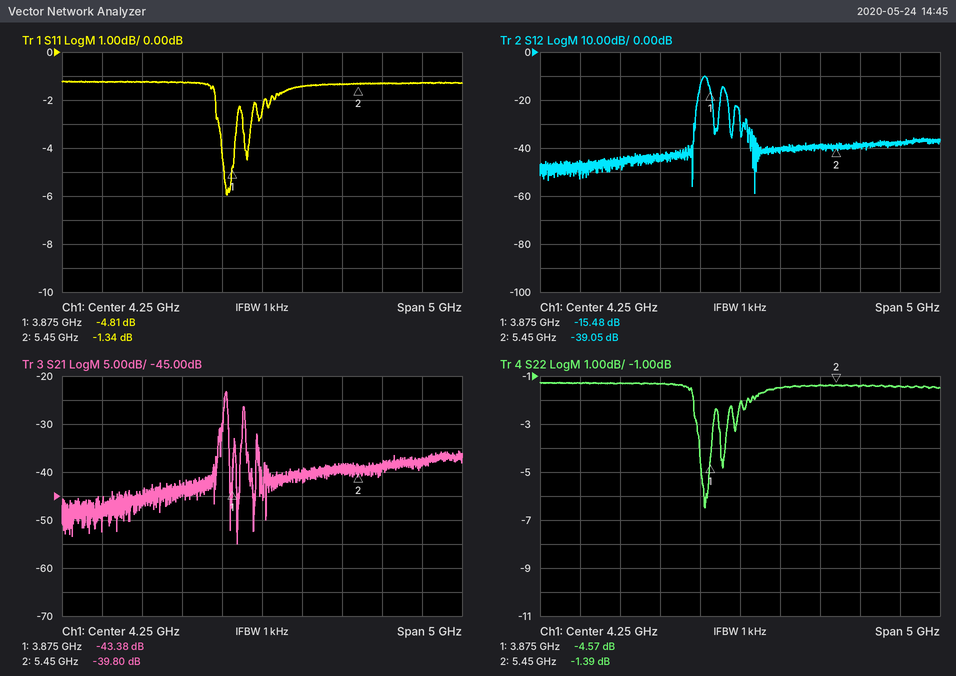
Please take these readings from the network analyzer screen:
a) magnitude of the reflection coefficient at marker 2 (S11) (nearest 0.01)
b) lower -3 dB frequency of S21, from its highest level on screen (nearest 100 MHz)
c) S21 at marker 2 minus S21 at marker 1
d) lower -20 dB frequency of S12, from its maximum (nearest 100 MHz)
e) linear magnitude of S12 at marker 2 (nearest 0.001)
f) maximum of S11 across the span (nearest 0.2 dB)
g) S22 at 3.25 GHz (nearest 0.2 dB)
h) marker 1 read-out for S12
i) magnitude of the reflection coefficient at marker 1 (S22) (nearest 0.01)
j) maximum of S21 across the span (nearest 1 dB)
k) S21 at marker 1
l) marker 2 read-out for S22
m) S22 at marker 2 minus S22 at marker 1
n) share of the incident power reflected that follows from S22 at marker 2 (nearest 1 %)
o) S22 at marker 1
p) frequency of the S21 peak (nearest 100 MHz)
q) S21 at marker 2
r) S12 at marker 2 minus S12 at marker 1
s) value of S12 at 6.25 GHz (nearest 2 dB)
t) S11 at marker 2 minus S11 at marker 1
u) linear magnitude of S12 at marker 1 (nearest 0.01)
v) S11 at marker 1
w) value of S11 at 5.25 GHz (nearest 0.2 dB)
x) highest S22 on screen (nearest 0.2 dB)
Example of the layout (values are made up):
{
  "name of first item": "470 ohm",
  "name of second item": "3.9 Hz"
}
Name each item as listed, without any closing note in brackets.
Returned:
{
  "magnitude of the reflection coefficient at marker 2 (S11)": "0.86",
  "lower -3 dB frequency of S21, from its highest level on screen": "3.8 GHz",
  "S21 at marker 2 minus S21 at marker 1": "3.58 dB",
  "lower -20 dB frequency of S12, from its maximum": "3.7 GHz",
  "linear magnitude of S12 at marker 2": "0.011",
  "maximum of S11 across the span": "-1.2 dB",
  "S22 at 3.25 GHz": "-1.4 dB",
  "marker 1 read-out for S12": "-15.48 dB",
  "magnitude of the reflection coefficient at marker 1 (S22)": "0.59",
  "maximum of S21 across the span": "-23 dB",
  "S21 at marker 1": "-43.38 dB",
  "marker 2 read-out for S22": "-1.39 dB",
  "S22 at marker 2 minus S22 at marker 1": "3.18 dB",
  "share of the incident power reflected that follows from S22 at marker 2": "73 %",
  "S22 at marker 1": "-4.57 dB",
  "frequency of the S21 peak": "3.8 GHz",
  "S21 at marker 2": "-39.80 dB",
  "S12 at marker 2 minus S12 at marker 1": "-23.57 dB",
  "value of S12 at 6.25 GHz": "-38 dB",
  "S11 at marker 2 minus S11 at marker 1": "3.47 dB",
  "linear magnitude of S12 at marker 1": "0.17",
  "S11 at marker 1": "-4.81 dB",
  "value of S11 at 5.25 GHz": "-1.4 dB",
  "highest S22 on screen": "-1.2 dB"
}
